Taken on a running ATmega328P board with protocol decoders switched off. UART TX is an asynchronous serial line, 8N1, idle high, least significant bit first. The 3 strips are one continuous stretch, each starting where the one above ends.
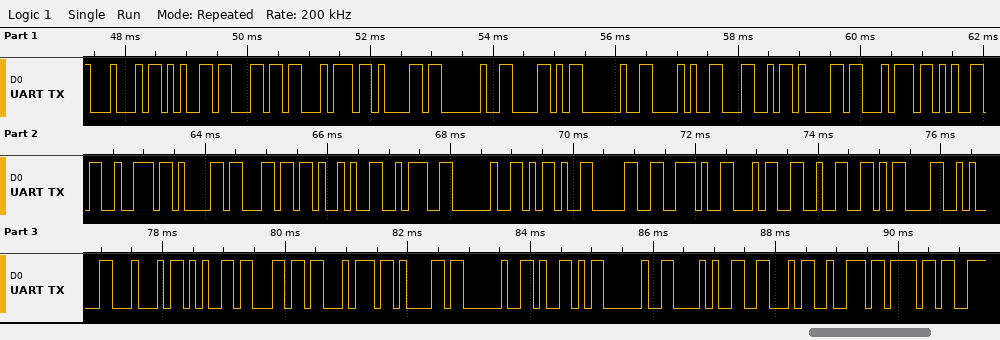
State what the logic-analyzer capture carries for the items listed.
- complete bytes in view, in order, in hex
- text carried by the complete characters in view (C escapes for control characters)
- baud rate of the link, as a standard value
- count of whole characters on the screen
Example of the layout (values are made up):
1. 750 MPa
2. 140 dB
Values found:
1. 44 65 6C 74 61 20 58 20 28 4C 61 74 65 72 61 6C 29 3A 20 2D 30 2E 34 32 0D 0A 44 65 6C 74 61 20 59 20 28 46 72 6F
2. "Delta X (Lateral): -0.42\r\nDelta Y (Fro"
3. 9600 baud
4. 38
